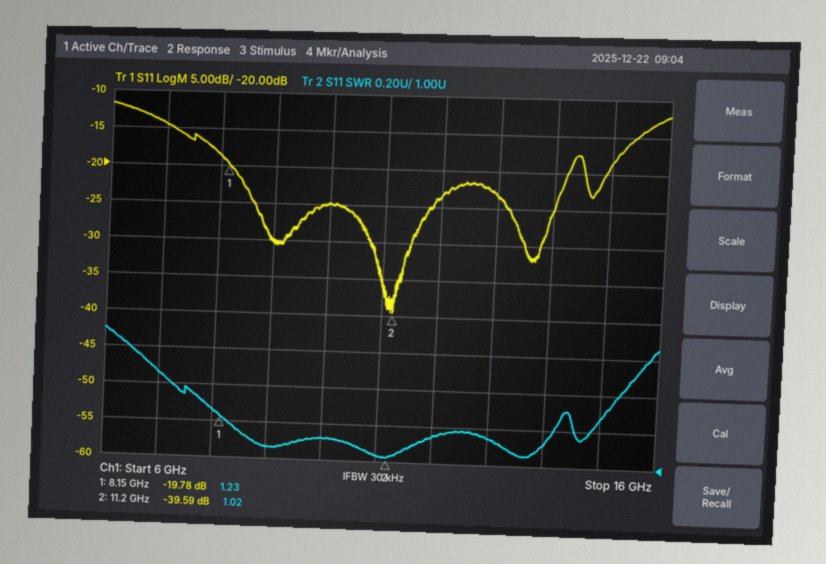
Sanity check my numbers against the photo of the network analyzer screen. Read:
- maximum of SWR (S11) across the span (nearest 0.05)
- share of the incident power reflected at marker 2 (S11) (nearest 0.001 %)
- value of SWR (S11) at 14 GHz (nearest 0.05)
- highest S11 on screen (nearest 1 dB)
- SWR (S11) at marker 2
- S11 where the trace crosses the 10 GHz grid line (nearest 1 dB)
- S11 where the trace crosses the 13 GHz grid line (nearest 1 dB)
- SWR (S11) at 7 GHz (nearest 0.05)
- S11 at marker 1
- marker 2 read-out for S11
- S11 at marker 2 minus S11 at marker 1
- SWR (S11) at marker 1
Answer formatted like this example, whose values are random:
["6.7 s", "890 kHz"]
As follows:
["1.70", "0.011 %", "1.10", "-12 dB", "1.02", "-25 dB", "-23 dB", "1.45", "-19.78 dB", "-39.59 dB", "-19.81 dB", "1.23"]
